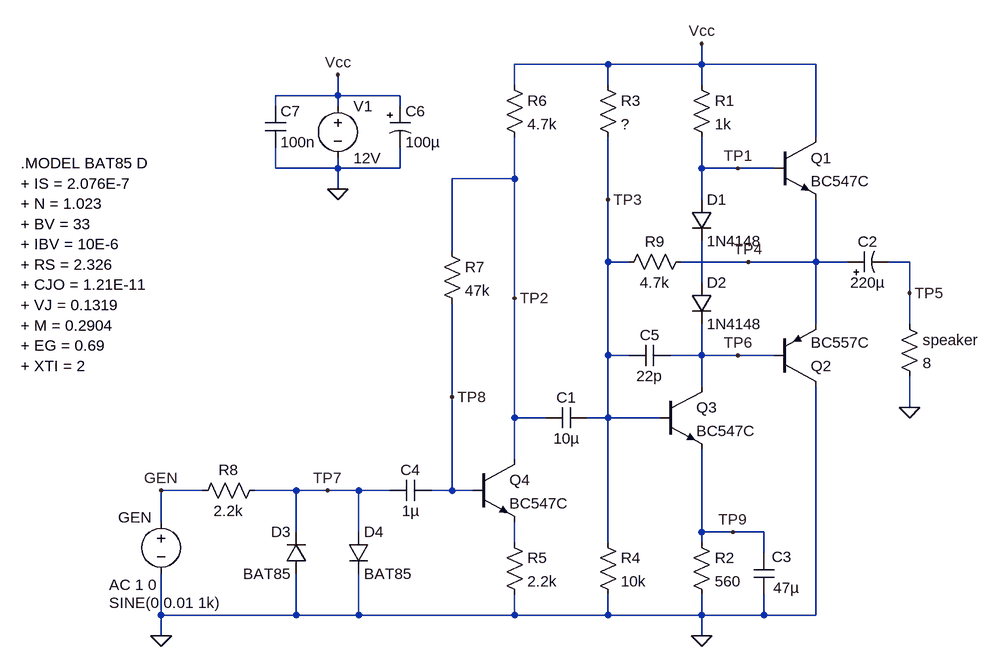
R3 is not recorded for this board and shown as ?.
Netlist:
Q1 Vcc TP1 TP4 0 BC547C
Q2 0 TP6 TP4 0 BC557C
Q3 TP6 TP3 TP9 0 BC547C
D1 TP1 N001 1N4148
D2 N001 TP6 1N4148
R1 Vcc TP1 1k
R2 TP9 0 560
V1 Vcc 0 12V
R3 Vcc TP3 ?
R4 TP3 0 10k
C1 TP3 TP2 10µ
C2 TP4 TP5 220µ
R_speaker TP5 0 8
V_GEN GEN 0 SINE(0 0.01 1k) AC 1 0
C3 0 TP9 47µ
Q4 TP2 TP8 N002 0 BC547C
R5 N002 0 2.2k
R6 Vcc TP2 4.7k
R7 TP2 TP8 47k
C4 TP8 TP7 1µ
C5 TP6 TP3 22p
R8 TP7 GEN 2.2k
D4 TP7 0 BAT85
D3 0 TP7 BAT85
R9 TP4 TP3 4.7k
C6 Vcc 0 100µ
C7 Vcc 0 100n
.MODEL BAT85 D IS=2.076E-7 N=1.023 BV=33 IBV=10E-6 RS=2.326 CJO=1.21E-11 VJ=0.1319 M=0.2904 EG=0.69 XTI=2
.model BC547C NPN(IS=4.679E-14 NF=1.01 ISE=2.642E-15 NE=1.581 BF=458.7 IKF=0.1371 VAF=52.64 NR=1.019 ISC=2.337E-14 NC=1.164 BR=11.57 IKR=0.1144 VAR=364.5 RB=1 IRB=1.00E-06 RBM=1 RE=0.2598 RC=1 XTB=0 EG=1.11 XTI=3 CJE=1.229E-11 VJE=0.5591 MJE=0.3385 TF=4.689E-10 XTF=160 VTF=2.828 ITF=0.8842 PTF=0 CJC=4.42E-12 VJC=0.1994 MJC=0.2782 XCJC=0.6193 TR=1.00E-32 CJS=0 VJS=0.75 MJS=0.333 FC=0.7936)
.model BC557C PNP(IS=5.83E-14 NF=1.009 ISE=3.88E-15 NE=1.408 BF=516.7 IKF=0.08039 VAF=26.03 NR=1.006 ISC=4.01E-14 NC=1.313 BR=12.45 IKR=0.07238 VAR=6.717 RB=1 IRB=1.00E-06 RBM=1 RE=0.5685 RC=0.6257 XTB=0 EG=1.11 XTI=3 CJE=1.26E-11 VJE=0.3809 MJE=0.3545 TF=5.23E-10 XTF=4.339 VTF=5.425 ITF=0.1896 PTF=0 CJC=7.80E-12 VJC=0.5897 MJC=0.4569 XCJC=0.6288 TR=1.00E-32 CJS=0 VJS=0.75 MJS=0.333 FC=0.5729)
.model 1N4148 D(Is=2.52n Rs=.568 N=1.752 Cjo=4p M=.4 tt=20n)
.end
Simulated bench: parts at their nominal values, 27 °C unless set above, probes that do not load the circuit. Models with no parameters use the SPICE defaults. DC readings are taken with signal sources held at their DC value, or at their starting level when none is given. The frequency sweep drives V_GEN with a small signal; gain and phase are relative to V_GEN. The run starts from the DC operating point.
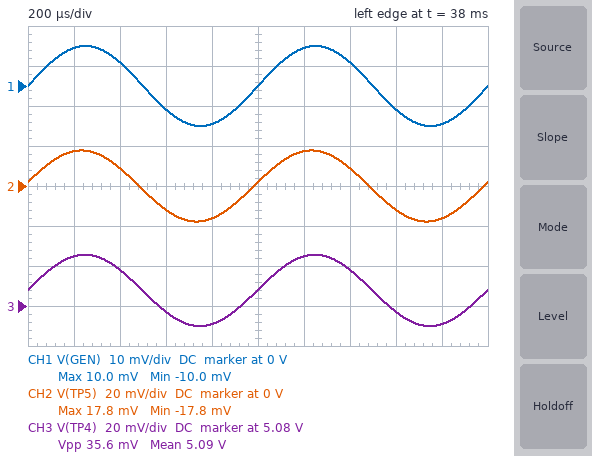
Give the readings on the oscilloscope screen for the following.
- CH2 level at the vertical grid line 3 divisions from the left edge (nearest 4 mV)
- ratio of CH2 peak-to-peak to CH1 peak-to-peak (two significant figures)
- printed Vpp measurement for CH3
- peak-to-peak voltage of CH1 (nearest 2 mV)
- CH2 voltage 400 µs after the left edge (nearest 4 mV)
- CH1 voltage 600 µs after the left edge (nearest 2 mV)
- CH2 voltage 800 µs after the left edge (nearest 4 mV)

-12 mV
1.8
35.6 mV
20 mV
8 mV
-6 mV
-16 mV
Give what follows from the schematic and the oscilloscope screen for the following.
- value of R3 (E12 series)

33 kΩ
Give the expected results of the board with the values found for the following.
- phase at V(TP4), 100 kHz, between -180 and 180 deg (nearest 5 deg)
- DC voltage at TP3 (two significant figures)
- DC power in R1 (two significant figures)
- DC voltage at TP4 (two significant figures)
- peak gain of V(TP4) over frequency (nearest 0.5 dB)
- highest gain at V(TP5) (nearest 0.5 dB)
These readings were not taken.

-10 deg
4.2 V
39 mW
5.1 V
5.0 dB
5.0 dB
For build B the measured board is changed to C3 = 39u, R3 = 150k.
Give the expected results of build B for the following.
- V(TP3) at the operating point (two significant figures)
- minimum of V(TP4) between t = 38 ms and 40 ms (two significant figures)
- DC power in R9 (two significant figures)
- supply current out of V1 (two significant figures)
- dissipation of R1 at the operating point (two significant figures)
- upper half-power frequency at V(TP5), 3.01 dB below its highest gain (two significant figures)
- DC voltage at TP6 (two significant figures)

3.9 V
5.5 V
580 µW
14 mA
33 mW
930 kHz
4.9 V
